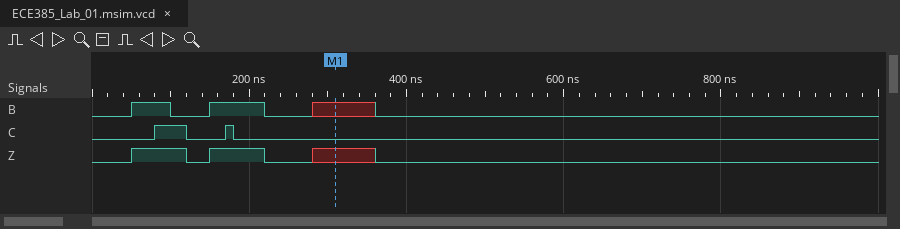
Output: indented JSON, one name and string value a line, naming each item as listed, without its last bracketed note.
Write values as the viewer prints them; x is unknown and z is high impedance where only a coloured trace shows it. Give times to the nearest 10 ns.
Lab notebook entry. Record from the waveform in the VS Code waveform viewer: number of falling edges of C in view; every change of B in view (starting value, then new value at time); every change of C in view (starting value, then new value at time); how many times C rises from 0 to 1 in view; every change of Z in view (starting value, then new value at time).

{
  "number of falling edges of C in view": "2",
  "every change of B in view": "0, 1 at 50 ns, 0 at 100 ns, 1 at 150 ns, 0 at 220 ns, x at 280 ns, 0 at 360 ns",
  "every change of C in view": "0, 1 at 80 ns, 0 at 120 ns, 1 at 170 ns, 0 at 180 ns",
  "how many times C rises from 0 to 1 in view": "2",
  "every change of Z in view": "0, 1 at 50 ns, 0 at 120 ns, 1 at 150 ns, 0 at 220 ns, x at 280 ns, 0 at 360 ns"
}
